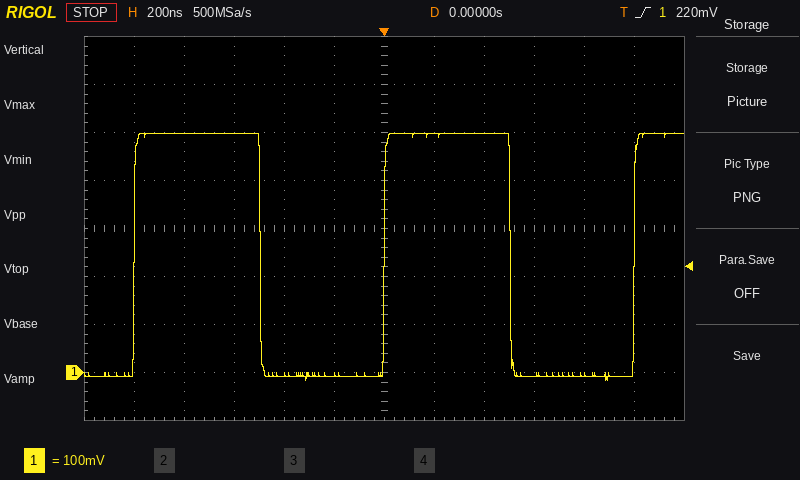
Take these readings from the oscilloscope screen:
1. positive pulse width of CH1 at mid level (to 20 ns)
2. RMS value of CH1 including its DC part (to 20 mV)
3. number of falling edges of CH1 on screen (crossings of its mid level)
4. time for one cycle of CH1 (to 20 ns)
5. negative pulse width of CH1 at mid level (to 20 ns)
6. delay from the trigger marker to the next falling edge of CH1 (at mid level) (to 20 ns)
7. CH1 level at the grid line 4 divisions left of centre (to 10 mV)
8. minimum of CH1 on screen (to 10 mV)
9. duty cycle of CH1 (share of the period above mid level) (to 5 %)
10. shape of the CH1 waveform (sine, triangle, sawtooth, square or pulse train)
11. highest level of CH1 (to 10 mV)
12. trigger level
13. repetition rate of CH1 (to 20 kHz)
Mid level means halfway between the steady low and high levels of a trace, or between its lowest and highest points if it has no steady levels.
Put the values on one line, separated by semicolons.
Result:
500 ns; 360 mV; 2; 1.00 µs; 500 ns; 500 ns; 500 mV; -20 mV; 50 %; square; 500 mV; 220 mV; 1.00 MHz
